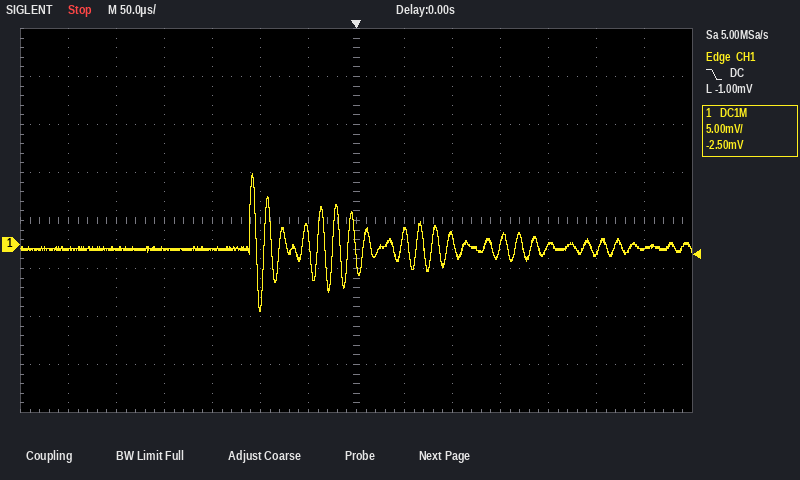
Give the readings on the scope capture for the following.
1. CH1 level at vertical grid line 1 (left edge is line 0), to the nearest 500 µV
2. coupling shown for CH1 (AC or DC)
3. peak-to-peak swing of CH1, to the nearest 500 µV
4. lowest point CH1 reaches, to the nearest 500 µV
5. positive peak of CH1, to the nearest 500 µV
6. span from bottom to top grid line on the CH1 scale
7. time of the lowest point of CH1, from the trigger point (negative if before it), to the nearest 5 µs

-500 µV
DC
14.5 mV
-7.0 mV
7.5 mV
40 mV
-100 µs
